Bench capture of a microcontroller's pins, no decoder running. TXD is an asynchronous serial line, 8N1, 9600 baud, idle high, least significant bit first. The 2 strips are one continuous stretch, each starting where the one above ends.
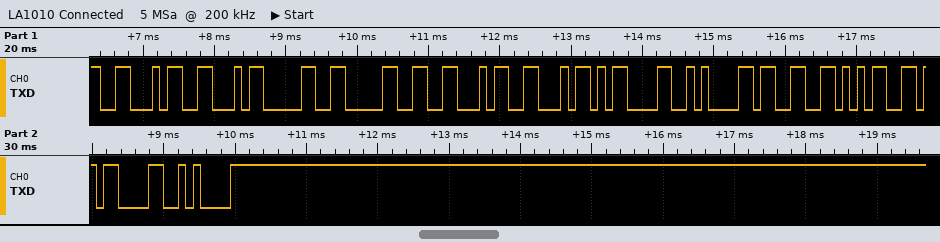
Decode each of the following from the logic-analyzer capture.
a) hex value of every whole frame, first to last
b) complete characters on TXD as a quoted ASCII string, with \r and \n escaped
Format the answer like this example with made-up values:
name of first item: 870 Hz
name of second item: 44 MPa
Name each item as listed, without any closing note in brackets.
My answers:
hex value of every whole frame, first to last: 0x46 0x46 0x30 0x30 0x46 0x46 0x0D 0x0A 0x33 0x35 0x0D 0x0A
complete characters on TXD as a quoted ASCII string, with \r and \n escaped: "FF00FF\r\n35\r\n"
